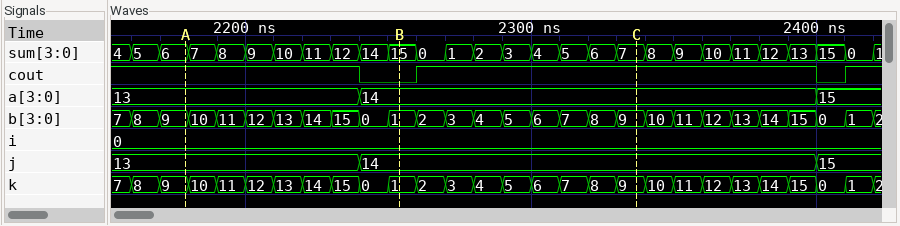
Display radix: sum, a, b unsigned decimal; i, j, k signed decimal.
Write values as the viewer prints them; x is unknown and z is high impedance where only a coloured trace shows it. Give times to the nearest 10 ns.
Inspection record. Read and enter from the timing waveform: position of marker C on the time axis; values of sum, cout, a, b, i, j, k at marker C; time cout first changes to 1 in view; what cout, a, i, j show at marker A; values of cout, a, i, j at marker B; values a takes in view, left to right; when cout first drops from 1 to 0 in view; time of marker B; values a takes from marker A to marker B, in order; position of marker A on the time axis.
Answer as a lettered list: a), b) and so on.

a) 2340 ns
b) sum=7, cout=1, a=14, b=9, i=0, j=14, k=9
c) 2260 ns
d) cout=1, a=13, i=0, j=13
e) cout=0, a=14, i=0, j=14
f) 13, 14, 15
g) 2240 ns
h) 2250 ns
i) 13, 14
j) 2180 ns
